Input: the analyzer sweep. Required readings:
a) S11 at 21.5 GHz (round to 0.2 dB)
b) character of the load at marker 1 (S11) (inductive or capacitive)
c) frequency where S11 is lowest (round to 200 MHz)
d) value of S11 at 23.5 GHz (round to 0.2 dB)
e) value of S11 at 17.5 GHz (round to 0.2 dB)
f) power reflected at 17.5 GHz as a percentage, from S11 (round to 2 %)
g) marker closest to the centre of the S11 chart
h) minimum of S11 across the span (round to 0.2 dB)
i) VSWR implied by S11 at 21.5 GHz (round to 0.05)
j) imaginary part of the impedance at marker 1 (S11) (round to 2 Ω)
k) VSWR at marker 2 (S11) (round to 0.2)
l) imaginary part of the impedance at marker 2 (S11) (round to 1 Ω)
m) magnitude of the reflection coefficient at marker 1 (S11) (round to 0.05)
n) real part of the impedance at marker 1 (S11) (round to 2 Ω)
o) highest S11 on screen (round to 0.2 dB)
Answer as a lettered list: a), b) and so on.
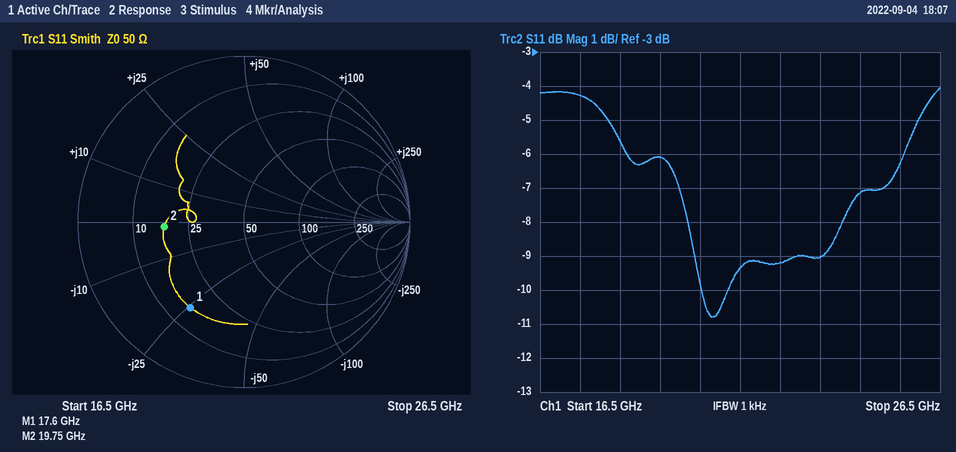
a) -9.4 dB
b) capacitive
c) 20.8 GHz
d) -9.0 dB
e) -4.2 dB
f) 38 %
g) marker 2
h) -10.8 dB
i) 2.05
j) -26 Ω
k) 2.8
l) -1 Ω
m) 0.60
n) 16 Ω
o) -4.0 dB
